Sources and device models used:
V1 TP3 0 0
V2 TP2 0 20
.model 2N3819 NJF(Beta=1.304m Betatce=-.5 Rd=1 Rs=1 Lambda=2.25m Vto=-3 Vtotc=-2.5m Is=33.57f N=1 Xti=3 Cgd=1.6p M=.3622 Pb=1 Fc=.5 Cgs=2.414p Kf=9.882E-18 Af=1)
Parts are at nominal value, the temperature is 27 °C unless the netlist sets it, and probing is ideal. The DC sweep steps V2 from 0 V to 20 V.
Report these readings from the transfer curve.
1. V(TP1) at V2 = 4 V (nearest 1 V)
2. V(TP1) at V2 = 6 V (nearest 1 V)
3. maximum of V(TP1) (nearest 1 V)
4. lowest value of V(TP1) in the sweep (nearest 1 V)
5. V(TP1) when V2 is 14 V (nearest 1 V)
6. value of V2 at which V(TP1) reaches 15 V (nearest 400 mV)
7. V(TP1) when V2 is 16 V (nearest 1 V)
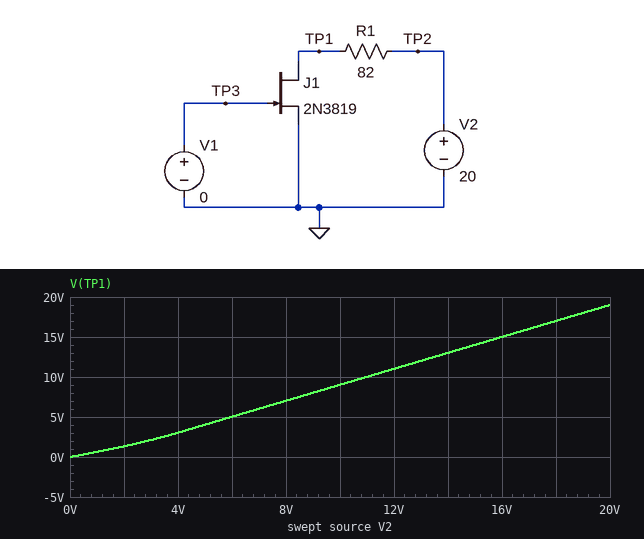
3 V
5 V
19 V
0 V
13 V
16.0 V
15 V
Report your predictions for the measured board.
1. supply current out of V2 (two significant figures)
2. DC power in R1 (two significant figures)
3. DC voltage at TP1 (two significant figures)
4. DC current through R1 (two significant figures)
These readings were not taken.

12 mA
12 mW
19 V
12 mA
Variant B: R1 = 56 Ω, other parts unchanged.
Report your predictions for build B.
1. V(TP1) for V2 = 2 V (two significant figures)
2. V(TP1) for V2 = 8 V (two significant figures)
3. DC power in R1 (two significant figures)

1.5 V
7.3 V
8.3 mW
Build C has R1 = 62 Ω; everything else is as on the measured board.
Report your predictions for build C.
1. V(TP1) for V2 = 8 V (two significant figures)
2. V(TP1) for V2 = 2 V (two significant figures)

7.3 V
1.5 V
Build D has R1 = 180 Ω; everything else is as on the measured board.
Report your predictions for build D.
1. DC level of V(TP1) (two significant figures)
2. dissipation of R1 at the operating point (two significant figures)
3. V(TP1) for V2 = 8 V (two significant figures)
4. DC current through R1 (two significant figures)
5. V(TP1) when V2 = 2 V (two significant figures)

18 V
26 mW
5.9 V
12 mA
920 mV
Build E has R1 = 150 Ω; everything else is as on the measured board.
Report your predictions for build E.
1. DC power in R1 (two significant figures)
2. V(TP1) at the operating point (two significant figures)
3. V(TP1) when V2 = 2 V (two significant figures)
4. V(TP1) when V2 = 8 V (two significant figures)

22 mW
18 V
1.0 V
6.2 V
